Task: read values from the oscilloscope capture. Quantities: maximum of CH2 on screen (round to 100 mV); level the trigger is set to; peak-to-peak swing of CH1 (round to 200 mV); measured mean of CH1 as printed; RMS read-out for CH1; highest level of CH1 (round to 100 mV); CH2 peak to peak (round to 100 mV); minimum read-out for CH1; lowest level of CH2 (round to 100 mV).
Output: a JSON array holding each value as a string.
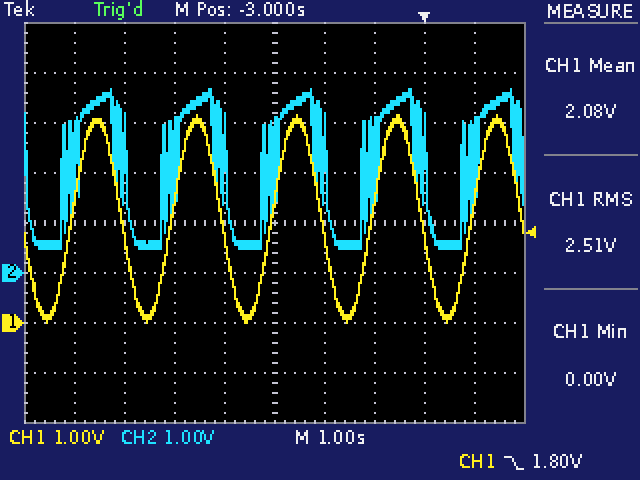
["3.7 V", "1.80 V", "4.2 V", "2.08 V", "2.51 V", "4.2 V", "3.2 V", "0.00 V", "500 mV"]
